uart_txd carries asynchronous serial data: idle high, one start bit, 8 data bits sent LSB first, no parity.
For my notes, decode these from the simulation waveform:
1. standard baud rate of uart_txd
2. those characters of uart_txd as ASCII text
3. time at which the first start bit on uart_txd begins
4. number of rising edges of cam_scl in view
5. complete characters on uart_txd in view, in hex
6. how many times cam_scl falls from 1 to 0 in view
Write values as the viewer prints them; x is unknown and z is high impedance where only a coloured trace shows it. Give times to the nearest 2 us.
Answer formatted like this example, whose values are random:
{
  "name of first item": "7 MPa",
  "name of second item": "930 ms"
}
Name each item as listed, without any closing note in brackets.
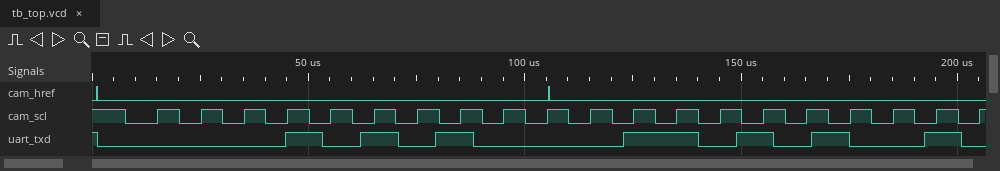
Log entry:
{
  "standard baud rate of uart_txd": "115200 baud",
  "those characters of uart_txd as ASCII text": "\"PX\"",
  "time at which the first start bit on uart_txd begins": "0 us",
  "number of rising edges of cam_scl in view": "20",
  "complete characters on uart_txd in view, in hex": "50, 58",
  "how many times cam_scl falls from 1 to 0 in view": "20"
}
